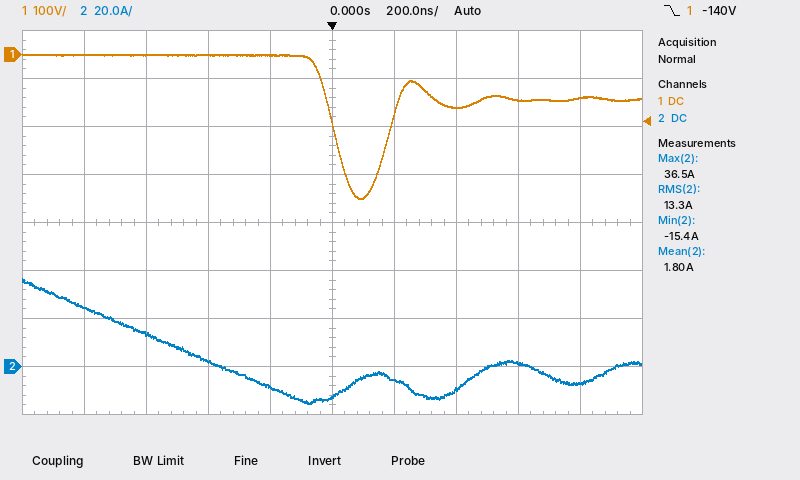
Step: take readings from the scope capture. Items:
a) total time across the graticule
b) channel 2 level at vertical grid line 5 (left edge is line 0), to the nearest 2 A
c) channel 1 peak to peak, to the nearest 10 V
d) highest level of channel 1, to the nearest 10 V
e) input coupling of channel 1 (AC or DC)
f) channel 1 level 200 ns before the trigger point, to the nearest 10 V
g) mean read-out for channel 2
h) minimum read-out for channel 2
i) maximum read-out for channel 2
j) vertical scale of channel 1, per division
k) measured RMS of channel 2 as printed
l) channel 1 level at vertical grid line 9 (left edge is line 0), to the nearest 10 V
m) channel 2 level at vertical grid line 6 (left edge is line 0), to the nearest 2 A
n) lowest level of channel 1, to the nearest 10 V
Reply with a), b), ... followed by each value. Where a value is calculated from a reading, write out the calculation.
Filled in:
a) 2 µs
b) -12 A
c) 0 V − (-300 V) = 300 V
d) 0 V
e) DC
f) 0 V
g) 1.80 A
h) -15.4 A
i) 36.5 A
j) 100 V
k) 13.3 A
l) -90 V
m) -6 A
n) -300 V
